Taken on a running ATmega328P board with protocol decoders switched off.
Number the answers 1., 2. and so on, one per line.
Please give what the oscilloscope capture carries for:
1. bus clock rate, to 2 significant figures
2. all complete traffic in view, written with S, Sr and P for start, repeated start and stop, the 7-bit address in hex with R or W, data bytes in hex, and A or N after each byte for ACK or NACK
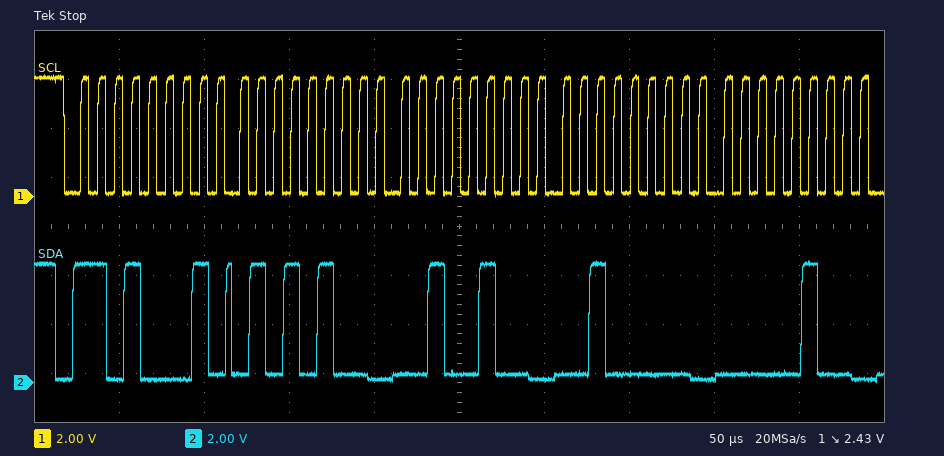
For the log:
1. 100 kHz
2. S 68R A 54 A 24 A 20 A 04 A
